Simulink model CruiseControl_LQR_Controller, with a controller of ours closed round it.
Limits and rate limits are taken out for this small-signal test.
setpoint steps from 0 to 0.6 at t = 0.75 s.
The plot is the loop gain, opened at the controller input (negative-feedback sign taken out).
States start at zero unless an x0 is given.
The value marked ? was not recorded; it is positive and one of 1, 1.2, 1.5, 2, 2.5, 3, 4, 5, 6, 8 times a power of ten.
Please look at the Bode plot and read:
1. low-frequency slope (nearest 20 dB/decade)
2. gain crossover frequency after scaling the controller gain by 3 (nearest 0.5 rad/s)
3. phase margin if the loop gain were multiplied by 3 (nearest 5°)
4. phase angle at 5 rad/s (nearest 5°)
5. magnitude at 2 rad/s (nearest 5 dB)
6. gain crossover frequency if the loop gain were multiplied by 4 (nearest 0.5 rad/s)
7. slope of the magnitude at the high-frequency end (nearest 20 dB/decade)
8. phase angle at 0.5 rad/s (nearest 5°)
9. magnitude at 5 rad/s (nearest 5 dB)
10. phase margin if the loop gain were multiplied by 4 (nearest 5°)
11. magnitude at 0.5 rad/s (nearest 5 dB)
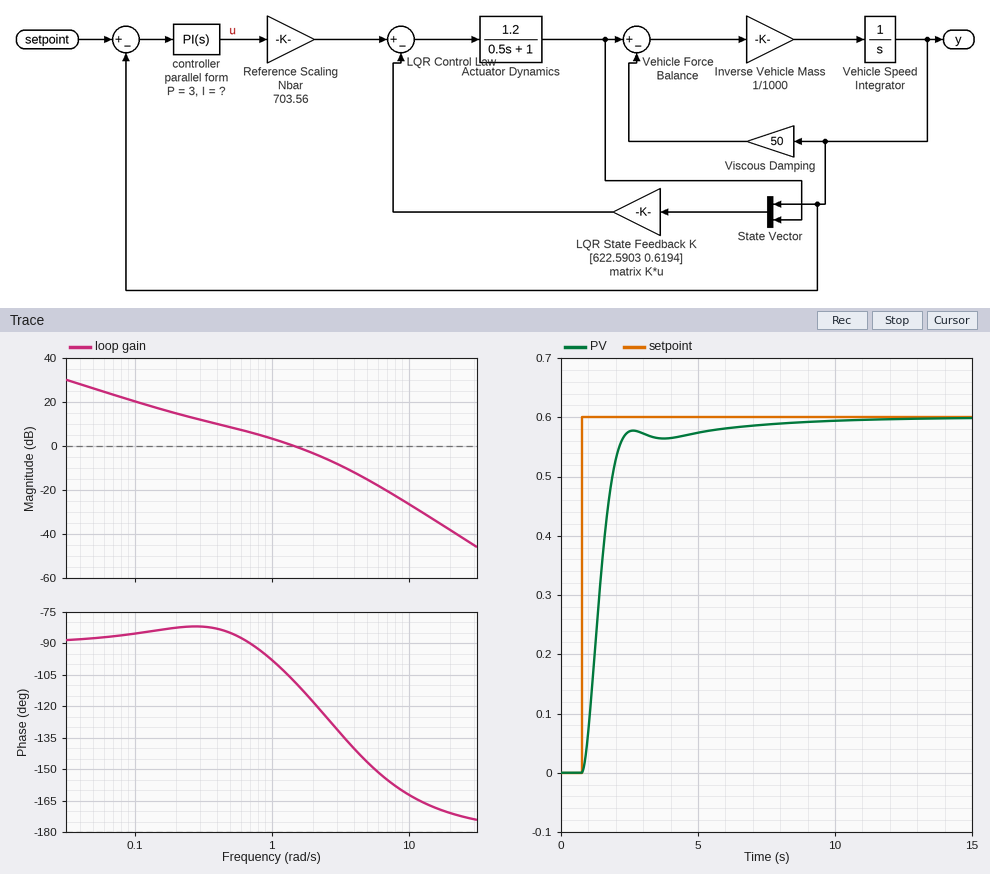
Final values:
-20 dB/decade
3.5 rad/s
45°
-145°
-5 dB
4.0 rad/s
-40 dB/decade
-85°
-15 dB
40°
10 dB
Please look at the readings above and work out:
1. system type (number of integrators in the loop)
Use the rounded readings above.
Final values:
1
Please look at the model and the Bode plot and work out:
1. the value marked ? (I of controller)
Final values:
1
